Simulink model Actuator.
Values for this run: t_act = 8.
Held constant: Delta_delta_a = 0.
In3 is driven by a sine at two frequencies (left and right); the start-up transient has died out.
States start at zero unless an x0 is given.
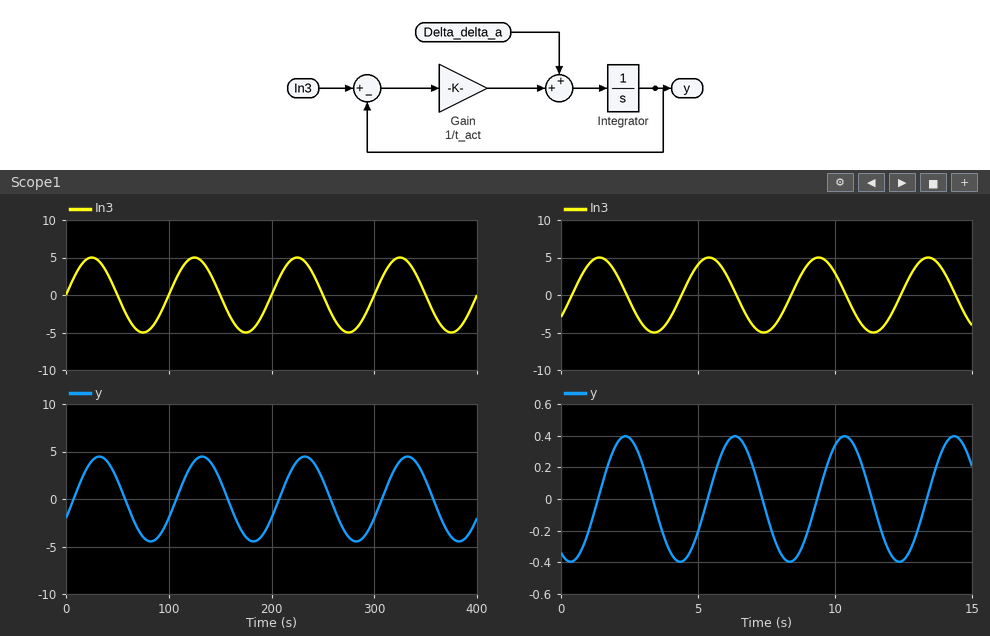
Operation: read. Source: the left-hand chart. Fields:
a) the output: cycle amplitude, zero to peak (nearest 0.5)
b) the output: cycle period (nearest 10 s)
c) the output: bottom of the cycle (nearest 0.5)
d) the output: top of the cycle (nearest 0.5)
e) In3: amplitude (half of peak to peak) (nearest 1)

4.5
100 s
-4.5
4.5
5
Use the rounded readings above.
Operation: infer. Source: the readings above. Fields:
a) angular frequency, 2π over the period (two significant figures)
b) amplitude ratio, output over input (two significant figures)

0.063 rad/s
0.90
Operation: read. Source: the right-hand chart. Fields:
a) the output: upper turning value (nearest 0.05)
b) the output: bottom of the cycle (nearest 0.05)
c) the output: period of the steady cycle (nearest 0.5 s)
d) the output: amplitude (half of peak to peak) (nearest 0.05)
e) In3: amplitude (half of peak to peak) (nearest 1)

0.40
-0.40
4.0 s
0.40
5
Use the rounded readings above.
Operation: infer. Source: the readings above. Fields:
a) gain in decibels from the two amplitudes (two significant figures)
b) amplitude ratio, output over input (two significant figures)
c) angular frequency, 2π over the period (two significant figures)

-22 dB
0.080
1.6 rad/s
